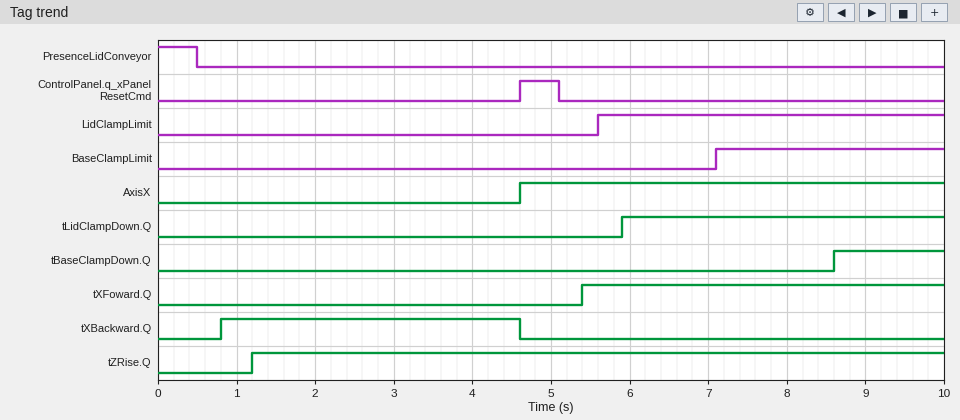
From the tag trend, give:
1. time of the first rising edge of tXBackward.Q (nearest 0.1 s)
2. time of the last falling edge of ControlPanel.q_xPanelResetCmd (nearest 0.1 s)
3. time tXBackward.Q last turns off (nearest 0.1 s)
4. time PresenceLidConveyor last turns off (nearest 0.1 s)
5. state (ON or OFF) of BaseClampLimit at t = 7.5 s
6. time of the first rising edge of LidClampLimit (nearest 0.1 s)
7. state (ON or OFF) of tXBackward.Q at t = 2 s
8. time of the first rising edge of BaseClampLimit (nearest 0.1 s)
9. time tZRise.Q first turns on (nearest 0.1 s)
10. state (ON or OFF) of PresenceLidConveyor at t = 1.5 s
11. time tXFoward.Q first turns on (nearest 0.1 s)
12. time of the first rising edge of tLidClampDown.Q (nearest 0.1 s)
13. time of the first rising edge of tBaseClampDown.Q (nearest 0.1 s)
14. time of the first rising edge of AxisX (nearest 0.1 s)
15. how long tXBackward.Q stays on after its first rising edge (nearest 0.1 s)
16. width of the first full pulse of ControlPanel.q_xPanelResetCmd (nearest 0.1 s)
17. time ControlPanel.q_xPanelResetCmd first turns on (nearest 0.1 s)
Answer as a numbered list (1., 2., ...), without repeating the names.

1. 0.8 s
2. 5.1 s
3. 4.6 s
4. 0.5 s
5. ON
6. 5.6 s
7. ON
8. 7.1 s
9. 1.2 s
10. OFF
11. 5.4 s
12. 5.9 s
13. 8.6 s
14. 4.6 s
15. 3.8 s
16. 0.5 s
17. 4.6 s
